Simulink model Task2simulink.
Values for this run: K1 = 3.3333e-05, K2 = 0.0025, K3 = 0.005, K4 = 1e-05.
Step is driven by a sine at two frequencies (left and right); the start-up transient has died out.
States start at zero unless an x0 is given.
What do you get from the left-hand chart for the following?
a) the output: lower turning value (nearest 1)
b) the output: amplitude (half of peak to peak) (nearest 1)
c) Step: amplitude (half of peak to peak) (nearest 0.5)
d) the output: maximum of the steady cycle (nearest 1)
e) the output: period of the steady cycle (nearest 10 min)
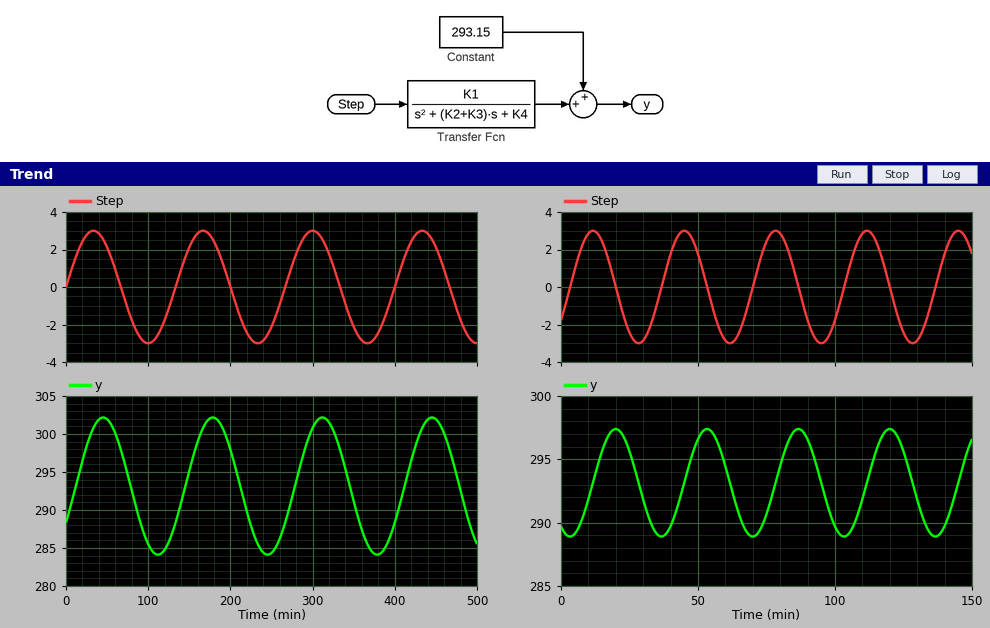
284
9
3.0
302
130 min
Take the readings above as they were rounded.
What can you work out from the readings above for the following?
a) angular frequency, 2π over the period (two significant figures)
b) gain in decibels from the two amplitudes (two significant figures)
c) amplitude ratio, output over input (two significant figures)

0.048 rad/min
9.5 dB
3.0
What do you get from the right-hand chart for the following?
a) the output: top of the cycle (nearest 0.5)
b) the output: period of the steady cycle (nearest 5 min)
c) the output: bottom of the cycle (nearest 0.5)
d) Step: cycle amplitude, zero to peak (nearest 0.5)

297.5
35 min
289.0
3.0
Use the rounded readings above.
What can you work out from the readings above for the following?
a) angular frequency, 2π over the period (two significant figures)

0.18 rad/min
